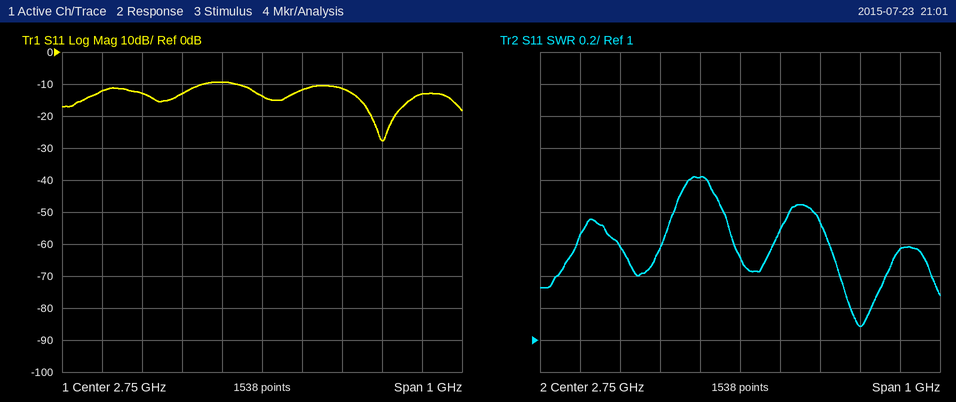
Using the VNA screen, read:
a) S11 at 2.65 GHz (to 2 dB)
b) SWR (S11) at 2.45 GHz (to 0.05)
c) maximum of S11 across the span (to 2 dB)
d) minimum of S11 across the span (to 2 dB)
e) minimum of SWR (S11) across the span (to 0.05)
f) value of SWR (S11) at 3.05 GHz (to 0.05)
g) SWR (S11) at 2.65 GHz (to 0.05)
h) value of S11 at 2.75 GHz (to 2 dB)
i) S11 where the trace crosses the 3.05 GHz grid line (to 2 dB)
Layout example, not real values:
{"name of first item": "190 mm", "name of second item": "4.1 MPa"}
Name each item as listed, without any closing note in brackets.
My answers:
{"S11 at 2.65 GHz": "-10 dB", "SWR (S11) at 2.45 GHz": "1.60", "maximum of S11 across the span": "-10 dB", "minimum of S11 across the span": "-28 dB", "minimum of SWR (S11) across the span": "1.10", "value of SWR (S11) at 3.05 GHz": "1.10", "SWR (S11) at 2.65 GHz": "2.00", "value of S11 at 2.75 GHz": "-14 dB", "S11 where the trace crosses the 3.05 GHz grid line": "-28 dB"}
